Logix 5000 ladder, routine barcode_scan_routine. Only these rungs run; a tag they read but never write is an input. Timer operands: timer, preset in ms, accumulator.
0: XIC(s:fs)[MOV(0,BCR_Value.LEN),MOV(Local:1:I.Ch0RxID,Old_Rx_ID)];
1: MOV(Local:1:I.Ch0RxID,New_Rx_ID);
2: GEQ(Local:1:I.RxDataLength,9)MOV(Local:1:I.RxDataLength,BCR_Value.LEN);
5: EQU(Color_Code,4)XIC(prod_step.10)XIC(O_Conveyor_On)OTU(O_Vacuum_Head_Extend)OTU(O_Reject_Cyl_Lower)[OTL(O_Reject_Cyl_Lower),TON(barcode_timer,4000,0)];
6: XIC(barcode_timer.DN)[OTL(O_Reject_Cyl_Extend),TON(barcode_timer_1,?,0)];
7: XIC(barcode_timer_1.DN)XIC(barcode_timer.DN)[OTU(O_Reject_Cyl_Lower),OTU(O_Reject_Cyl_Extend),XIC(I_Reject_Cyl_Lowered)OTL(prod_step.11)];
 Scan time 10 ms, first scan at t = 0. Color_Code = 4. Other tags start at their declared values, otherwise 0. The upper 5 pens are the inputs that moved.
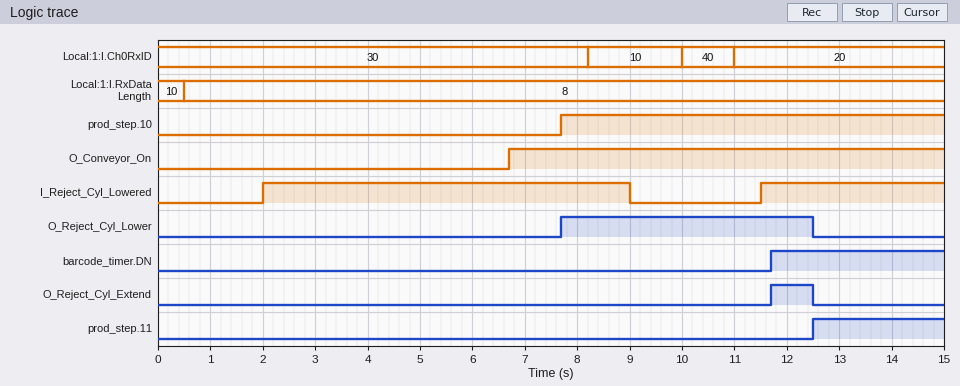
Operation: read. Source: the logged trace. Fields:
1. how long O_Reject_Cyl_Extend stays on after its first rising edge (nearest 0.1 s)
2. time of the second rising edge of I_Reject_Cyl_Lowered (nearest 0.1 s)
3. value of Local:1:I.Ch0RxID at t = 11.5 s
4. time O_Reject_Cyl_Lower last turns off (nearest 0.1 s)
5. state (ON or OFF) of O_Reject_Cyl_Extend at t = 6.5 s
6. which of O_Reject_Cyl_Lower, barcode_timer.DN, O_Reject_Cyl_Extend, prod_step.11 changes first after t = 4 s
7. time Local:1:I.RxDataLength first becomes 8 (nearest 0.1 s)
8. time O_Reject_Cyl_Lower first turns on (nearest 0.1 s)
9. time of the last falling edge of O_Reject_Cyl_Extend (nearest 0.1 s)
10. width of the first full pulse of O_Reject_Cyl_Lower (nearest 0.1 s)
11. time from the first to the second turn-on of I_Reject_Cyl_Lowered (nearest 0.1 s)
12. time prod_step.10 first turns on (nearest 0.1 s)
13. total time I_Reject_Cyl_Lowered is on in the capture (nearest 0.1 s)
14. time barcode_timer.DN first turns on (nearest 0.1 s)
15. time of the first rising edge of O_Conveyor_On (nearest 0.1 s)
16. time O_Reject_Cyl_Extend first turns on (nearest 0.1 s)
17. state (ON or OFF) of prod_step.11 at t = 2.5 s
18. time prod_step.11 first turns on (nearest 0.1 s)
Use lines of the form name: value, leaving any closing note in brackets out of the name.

how long O_Reject_Cyl_Extend stays on after its first rising edge: 0.8 s
time of the second rising edge of I_Reject_Cyl_Lowered: 11.5 s
value of Local:1:I.Ch0RxID at t = 11.5 s: 20
time O_Reject_Cyl_Lower last turns off: 12.5 s
state (ON or OFF) of O_Reject_Cyl_Extend at t = 6.5 s: OFF
which of O_Reject_Cyl_Lower, barcode_timer.DN, O_Reject_Cyl_Extend, prod_step.11 changes first after t = 4 s: O_Reject_Cyl_Lower
time Local:1:I.RxDataLength first becomes 8: 0.5 s
time O_Reject_Cyl_Lower first turns on: 7.7 s
time of the last falling edge of O_Reject_Cyl_Extend: 12.5 s
width of the first full pulse of O_Reject_Cyl_Lower: 4.8 s
time from the first to the second turn-on of I_Reject_Cyl_Lowered: 9.5 s
time prod_step.10 first turns on: 7.7 s
total time I_Reject_Cyl_Lowered is on in the capture: 10.5 s
time barcode_timer.DN first turns on: 11.7 s
time of the first rising edge of O_Conveyor_On: 6.7 s
time O_Reject_Cyl_Extend first turns on: 11.7 s
state (ON or OFF) of prod_step.11 at t = 2.5 s: OFF
time prod_step.11 first turns on: 12.5 s
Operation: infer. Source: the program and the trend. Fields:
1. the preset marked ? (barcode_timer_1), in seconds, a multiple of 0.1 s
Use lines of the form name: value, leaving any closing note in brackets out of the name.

the preset marked ? (barcode_timer_1), in seconds, a multiple of 0.1 s: 0.8 s
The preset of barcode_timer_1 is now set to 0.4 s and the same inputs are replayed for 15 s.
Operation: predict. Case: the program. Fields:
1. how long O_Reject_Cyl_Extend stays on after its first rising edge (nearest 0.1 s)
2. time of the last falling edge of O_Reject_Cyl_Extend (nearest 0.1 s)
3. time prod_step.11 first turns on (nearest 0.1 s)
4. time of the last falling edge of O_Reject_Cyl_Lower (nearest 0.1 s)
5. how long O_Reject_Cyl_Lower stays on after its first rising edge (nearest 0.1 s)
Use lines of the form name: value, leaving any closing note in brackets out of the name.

how long O_Reject_Cyl_Extend stays on after its first rising edge: 0.4 s
time of the last falling edge of O_Reject_Cyl_Extend: 12.1 s
time prod_step.11 first turns on: 12.1 s
time of the last falling edge of O_Reject_Cyl_Lower: 12.1 s
how long O_Reject_Cyl_Lower stays on after its first rising edge: 4.4 s
